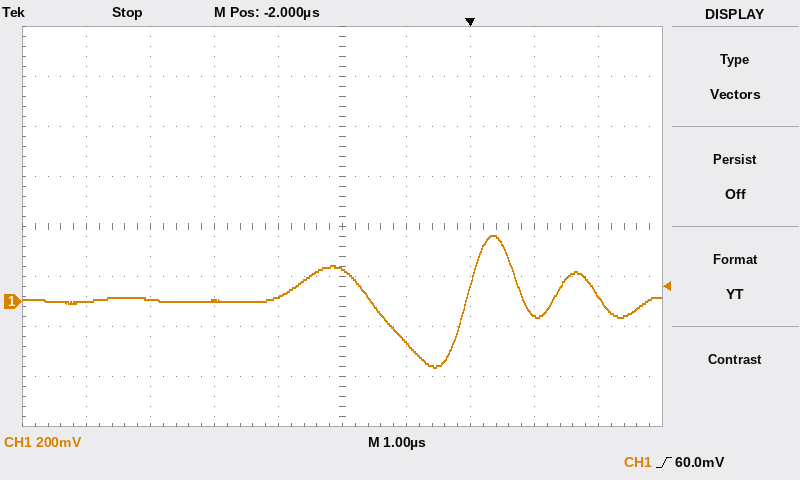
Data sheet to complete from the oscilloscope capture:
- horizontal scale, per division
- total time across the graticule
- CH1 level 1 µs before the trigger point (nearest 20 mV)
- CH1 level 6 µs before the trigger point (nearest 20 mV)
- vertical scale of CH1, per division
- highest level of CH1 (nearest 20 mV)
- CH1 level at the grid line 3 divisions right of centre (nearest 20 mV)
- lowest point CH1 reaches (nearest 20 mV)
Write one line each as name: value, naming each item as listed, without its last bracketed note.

horizontal scale, per division: 1 µs
total time across the graticule: 10 µs
CH1 level 1 µs before the trigger point: -160 mV
CH1 level 6 µs before the trigger point: 0 mV
vertical scale of CH1, per division: 200 mV
highest level of CH1: 260 mV
CH1 level at the grid line 3 divisions right of centre: -60 mV
lowest point CH1 reaches: -260 mV
